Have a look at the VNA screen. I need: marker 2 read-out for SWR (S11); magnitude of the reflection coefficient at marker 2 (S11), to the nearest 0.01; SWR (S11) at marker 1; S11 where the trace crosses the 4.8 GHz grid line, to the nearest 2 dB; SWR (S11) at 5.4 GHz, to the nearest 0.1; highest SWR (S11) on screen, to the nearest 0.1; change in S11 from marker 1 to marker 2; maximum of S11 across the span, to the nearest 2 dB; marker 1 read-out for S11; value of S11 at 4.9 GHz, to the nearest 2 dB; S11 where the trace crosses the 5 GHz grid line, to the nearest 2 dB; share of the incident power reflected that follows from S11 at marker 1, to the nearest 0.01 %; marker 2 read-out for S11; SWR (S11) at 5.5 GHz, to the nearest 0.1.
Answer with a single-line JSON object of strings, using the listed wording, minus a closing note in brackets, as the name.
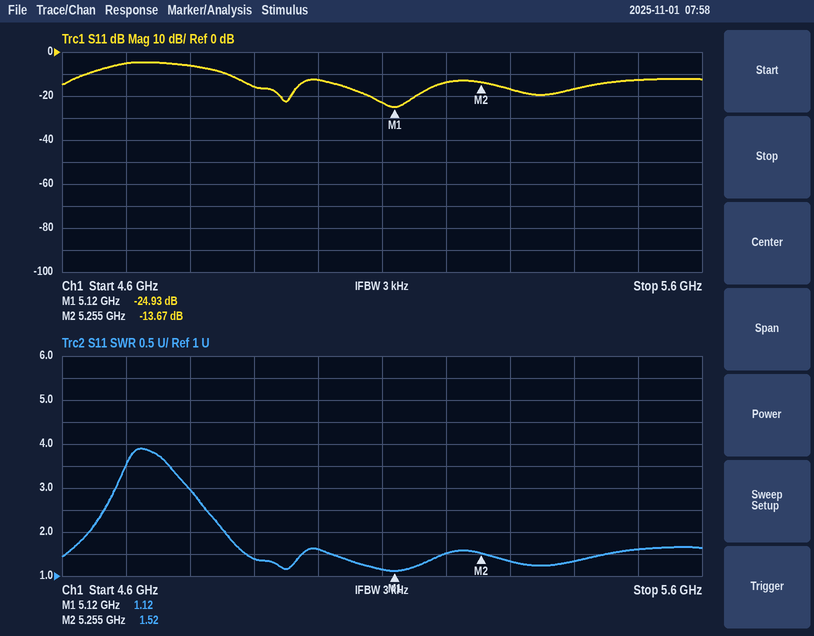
{"marker 2 read-out for SWR": "1.52", "magnitude of the reflection coefficient at marker 2 (S11), to the nearest 0.01": "0.21", "SWR (S11) at marker 1": "1.12", "S11 where the trace crosses the 4.8 GHz grid line, to the nearest 2 dB": "-6 dB", "SWR (S11) at 5.4 GHz, to the nearest 0.1": "1.3", "highest SWR (S11) on screen, to the nearest 0.1": "3.9", "change in S11 from marker 1 to marker 2": "11.26 dB", "maximum of S11 across the span, to the nearest 2 dB": "-4 dB", "marker 1 read-out for S11": "-24.93 dB", "value of S11 at 4.9 GHz, to the nearest 2 dB": "-16 dB", "S11 where the trace crosses the 5 GHz grid line, to the nearest 2 dB": "-12 dB", "share of the incident power reflected that follows from S11 at marker 1, to the nearest 0.01 %": "0.32 %", "marker 2 read-out for S11": "-13.67 dB", "SWR (S11) at 5.5 GHz, to the nearest 0.1": "1.6"}
